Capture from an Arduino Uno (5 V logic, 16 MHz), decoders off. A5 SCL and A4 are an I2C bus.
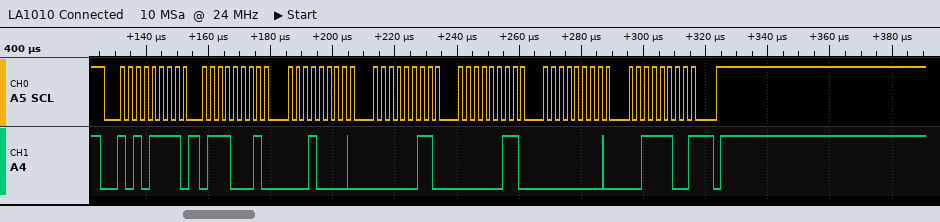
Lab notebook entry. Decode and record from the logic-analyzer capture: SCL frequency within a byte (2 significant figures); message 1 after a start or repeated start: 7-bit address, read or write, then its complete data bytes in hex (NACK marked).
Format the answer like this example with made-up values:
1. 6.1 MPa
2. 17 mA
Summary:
1. 400 kHz
2. 0x57 read: 71 10 03 03 00 3C NACK
